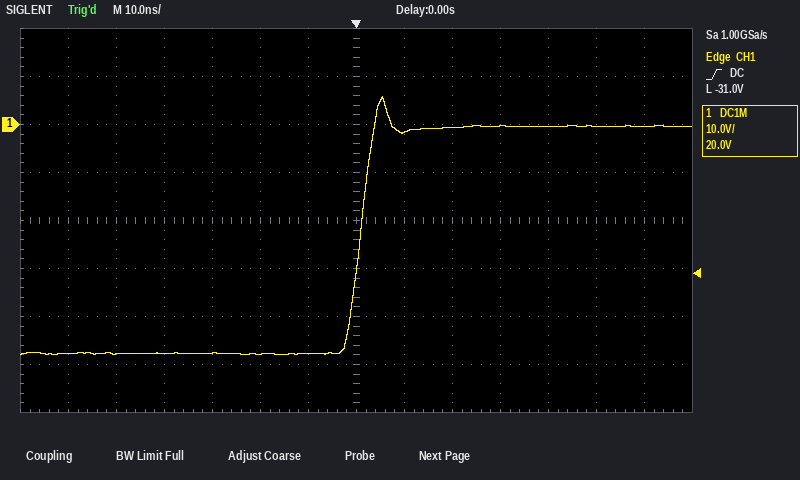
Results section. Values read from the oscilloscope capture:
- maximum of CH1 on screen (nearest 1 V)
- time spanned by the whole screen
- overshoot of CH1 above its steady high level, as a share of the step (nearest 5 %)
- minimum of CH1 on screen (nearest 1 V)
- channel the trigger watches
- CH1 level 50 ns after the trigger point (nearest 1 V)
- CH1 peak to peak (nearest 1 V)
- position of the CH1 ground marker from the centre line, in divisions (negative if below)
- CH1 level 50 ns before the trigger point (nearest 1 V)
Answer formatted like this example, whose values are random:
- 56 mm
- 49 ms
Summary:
- 6 V
- 140 ns
- 15 %
- -48 V
- CH1
- 0 V
- 54 V
- +2.0 div
- -48 V
